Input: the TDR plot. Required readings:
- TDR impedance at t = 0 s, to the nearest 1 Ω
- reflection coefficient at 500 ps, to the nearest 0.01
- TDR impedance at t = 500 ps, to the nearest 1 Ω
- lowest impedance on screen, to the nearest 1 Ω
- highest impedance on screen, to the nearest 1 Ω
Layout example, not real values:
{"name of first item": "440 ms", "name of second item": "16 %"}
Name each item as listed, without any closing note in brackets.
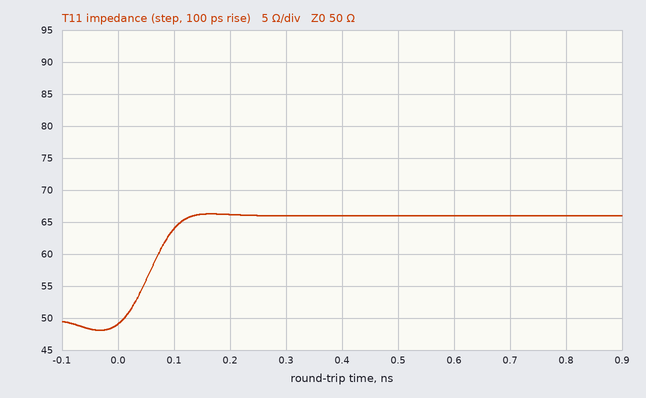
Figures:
{"TDR impedance at t = 0 s, to the nearest 1 Ω": "49 Ω", "reflection coefficient at 500 ps, to the nearest 0.01": "+0.14", "TDR impedance at t = 500 ps, to the nearest 1 Ω": "66 Ω", "lowest impedance on screen, to the nearest 1 Ω": "48 Ω", "highest impedance on screen, to the nearest 1 Ω": "66 Ω"}
